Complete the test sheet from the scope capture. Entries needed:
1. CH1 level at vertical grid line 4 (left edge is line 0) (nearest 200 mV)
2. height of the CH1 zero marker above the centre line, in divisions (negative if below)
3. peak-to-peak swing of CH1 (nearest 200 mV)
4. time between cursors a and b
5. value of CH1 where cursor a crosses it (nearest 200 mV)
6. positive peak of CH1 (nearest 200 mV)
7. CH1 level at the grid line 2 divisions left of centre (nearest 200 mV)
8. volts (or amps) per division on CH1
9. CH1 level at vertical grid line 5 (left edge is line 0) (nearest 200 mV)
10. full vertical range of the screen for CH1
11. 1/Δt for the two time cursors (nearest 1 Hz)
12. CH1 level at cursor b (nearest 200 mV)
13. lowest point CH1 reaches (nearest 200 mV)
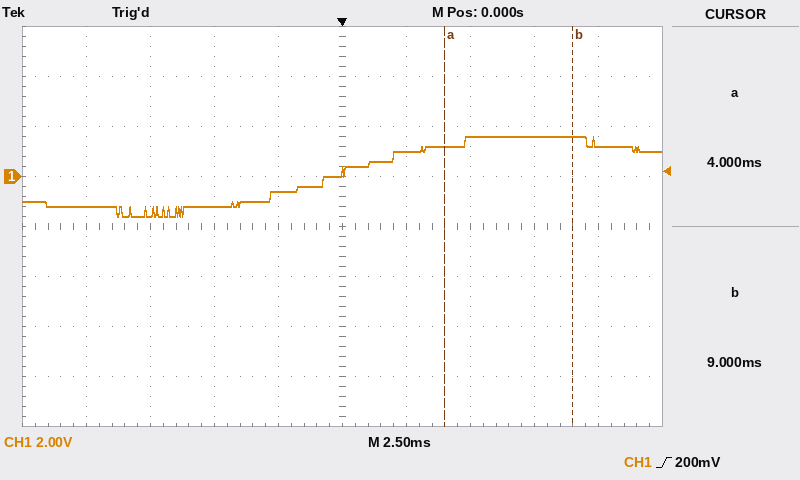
-600 mV
+1.0 div
3.2 V
5.00 ms
1.2 V
1.6 V
-1.2 V
2 V
200 mV
16 V
200 Hz
1.6 V
-1.6 V
